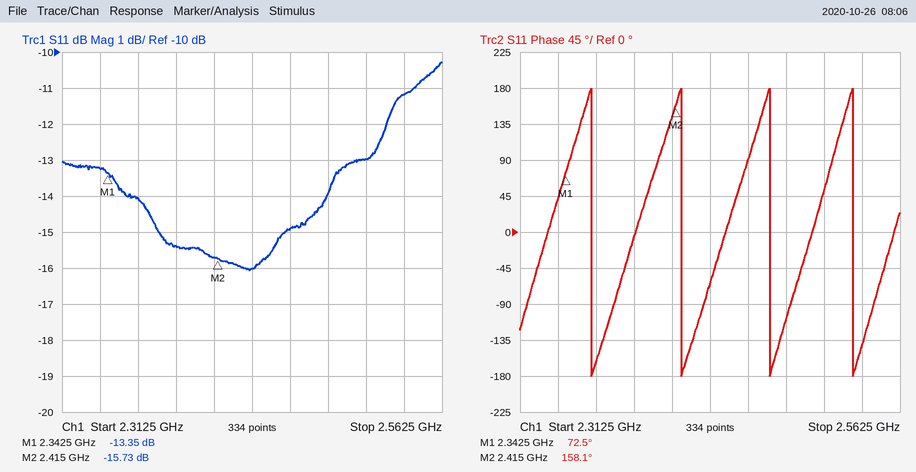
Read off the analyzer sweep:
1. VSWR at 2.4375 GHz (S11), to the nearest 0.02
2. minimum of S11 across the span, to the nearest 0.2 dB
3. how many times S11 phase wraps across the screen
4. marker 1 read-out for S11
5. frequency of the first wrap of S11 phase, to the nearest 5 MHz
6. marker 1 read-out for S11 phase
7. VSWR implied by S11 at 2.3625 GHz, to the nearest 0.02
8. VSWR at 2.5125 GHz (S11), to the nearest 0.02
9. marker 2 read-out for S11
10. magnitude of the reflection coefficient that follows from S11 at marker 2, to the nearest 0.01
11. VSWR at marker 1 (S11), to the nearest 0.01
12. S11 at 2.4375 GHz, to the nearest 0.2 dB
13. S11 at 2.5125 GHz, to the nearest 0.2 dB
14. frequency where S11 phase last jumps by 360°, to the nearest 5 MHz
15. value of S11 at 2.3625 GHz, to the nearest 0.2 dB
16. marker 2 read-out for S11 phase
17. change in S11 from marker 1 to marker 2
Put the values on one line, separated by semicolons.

1.38; -16.0 dB; 4; -13.35 dB; 2.360 GHz; 72.5°; 1.50; 1.58; -15.73 dB; 0.16; 1.55; -16.0 dB; -13.0 dB; 2.530 GHz; -14.0 dB; 158.1°; -2.38 dB
